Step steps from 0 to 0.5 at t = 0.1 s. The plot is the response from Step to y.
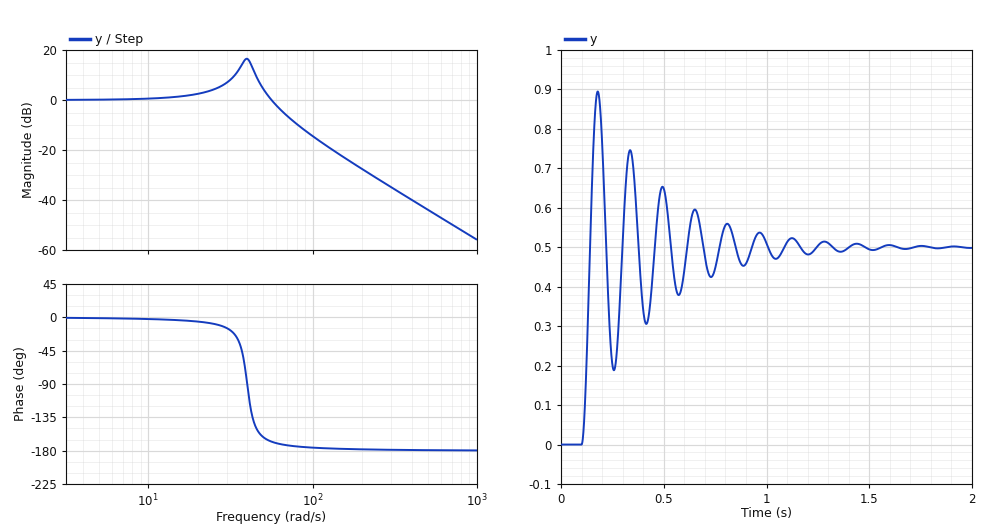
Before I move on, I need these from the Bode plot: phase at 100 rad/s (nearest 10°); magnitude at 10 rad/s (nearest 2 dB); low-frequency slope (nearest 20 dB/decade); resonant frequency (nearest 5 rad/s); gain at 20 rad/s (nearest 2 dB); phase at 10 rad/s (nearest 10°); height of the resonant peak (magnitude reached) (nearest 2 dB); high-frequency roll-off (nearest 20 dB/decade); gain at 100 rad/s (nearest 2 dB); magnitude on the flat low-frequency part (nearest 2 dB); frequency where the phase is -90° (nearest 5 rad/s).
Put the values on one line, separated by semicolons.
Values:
-180°; 0 dB; 0 dB/decade; 40 rad/s; 2 dB; 0°; 16 dB; -40 dB/decade; -14 dB; 0 dB; 40 rad/s
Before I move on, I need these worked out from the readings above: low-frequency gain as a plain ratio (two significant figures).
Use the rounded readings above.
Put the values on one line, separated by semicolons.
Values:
1.0
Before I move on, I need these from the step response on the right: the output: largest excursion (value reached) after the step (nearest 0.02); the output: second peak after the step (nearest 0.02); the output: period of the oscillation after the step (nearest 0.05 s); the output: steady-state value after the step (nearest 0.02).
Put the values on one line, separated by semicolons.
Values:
0.90; 0.74; 0.15 s; 0.50
